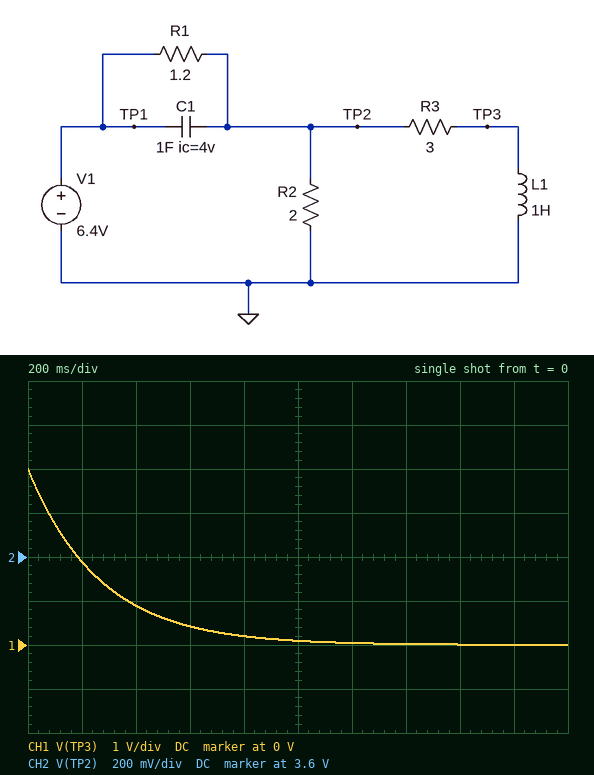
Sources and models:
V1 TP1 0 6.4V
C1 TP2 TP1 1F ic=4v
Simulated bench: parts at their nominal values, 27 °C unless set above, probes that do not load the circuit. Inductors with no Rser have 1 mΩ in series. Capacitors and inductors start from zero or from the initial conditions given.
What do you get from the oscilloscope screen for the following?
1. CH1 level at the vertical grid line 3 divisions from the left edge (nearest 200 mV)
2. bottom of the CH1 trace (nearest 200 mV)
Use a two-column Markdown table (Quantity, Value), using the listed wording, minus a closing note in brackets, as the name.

| Quantity | Value |
|---|---|
| CH1 level at the vertical grid line 3 divisions from the left edge | 400 mV |
| bottom of the CH1 trace | 0 V |
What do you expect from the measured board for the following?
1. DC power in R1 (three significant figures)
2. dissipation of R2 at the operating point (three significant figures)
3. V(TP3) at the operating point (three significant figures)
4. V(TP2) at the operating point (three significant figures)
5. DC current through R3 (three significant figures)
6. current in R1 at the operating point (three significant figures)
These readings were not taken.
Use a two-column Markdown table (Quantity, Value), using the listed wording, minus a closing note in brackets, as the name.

| Quantity | Value |
|---|---|
| DC power in R1 | 8.53 W |
| dissipation of R2 at the operating point | 5.12 W |
| V(TP3) at the operating point | 1.07 mV |
| V(TP2) at the operating point | 3.20 V |
| DC current through R3 | 1.07 A |
| current in R1 at the operating point | 2.67 A |
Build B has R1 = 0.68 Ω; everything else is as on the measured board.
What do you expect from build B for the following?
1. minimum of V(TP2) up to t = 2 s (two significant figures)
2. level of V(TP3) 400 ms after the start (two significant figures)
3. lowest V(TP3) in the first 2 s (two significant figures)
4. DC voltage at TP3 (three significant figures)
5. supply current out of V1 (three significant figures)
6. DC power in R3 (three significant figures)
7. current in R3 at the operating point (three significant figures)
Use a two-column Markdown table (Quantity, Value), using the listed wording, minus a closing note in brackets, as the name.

| Quantity | Value |
|---|---|
| minimum of V(TP2) up to t = 2 s | 4.1 V |
| level of V(TP3) 400 ms after the start | 1.2 V |
| lowest V(TP3) in the first 2 s | 5.6 mV |
| DC voltage at TP3 | 1.36 mV |
| supply current out of V1 | 3.40 A |
| DC power in R3 | 5.56 W |
| current in R3 at the operating point | 1.36 A |
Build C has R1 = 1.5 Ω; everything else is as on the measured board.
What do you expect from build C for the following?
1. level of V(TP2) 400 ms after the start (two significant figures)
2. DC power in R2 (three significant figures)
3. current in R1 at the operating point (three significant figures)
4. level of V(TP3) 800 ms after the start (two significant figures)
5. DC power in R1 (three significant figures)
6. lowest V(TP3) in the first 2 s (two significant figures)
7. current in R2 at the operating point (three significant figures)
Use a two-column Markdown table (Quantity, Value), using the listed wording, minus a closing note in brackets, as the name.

| Quantity | Value |
|---|---|
| level of V(TP2) 400 ms after the start | 3.0 V |
| DC power in R2 | 4.05 W |
| current in R1 at the operating point | 2.37 A |
| level of V(TP3) 800 ms after the start | 170 mV |
| DC power in R1 | 8.43 W |
| lowest V(TP3) in the first 2 s | 2.6 mV |
| current in R2 at the operating point | 1.42 A |
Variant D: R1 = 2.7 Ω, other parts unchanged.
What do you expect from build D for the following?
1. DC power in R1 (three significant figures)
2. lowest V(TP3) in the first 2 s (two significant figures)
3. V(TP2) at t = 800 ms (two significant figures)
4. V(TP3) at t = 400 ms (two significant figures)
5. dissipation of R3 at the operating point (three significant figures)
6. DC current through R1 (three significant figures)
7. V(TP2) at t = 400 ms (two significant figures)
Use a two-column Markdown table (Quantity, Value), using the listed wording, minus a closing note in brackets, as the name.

| Quantity | Value |
|---|---|
| DC power in R1 | 7.27 W |
| lowest V(TP3) in the first 2 s | 1.3 mV |
| V(TP2) at t = 800 ms | 2.0 V |
| V(TP3) at t = 400 ms | 520 mV |
| dissipation of R3 at the operating point | 1.29 W |
| DC current through R1 | 1.64 A |
| V(TP2) at t = 400 ms | 2.1 V |
